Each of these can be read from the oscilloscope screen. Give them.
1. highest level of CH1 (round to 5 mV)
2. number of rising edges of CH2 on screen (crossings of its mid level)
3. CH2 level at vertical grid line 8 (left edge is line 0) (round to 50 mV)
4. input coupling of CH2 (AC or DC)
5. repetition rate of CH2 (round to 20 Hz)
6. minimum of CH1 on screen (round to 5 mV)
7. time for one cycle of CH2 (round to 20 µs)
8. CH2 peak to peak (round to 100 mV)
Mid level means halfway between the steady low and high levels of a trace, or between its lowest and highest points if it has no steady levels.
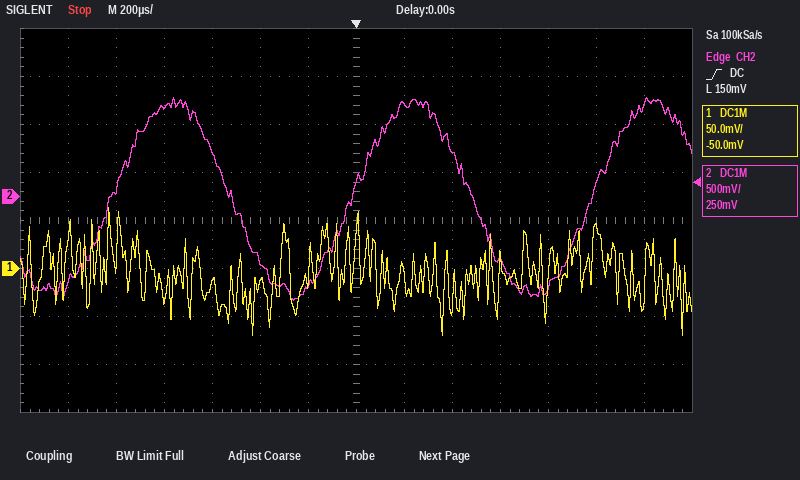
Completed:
65 mV
3
950 mV
DC
1.00 kHz
-70 mV
1.00 ms
2.10 V
